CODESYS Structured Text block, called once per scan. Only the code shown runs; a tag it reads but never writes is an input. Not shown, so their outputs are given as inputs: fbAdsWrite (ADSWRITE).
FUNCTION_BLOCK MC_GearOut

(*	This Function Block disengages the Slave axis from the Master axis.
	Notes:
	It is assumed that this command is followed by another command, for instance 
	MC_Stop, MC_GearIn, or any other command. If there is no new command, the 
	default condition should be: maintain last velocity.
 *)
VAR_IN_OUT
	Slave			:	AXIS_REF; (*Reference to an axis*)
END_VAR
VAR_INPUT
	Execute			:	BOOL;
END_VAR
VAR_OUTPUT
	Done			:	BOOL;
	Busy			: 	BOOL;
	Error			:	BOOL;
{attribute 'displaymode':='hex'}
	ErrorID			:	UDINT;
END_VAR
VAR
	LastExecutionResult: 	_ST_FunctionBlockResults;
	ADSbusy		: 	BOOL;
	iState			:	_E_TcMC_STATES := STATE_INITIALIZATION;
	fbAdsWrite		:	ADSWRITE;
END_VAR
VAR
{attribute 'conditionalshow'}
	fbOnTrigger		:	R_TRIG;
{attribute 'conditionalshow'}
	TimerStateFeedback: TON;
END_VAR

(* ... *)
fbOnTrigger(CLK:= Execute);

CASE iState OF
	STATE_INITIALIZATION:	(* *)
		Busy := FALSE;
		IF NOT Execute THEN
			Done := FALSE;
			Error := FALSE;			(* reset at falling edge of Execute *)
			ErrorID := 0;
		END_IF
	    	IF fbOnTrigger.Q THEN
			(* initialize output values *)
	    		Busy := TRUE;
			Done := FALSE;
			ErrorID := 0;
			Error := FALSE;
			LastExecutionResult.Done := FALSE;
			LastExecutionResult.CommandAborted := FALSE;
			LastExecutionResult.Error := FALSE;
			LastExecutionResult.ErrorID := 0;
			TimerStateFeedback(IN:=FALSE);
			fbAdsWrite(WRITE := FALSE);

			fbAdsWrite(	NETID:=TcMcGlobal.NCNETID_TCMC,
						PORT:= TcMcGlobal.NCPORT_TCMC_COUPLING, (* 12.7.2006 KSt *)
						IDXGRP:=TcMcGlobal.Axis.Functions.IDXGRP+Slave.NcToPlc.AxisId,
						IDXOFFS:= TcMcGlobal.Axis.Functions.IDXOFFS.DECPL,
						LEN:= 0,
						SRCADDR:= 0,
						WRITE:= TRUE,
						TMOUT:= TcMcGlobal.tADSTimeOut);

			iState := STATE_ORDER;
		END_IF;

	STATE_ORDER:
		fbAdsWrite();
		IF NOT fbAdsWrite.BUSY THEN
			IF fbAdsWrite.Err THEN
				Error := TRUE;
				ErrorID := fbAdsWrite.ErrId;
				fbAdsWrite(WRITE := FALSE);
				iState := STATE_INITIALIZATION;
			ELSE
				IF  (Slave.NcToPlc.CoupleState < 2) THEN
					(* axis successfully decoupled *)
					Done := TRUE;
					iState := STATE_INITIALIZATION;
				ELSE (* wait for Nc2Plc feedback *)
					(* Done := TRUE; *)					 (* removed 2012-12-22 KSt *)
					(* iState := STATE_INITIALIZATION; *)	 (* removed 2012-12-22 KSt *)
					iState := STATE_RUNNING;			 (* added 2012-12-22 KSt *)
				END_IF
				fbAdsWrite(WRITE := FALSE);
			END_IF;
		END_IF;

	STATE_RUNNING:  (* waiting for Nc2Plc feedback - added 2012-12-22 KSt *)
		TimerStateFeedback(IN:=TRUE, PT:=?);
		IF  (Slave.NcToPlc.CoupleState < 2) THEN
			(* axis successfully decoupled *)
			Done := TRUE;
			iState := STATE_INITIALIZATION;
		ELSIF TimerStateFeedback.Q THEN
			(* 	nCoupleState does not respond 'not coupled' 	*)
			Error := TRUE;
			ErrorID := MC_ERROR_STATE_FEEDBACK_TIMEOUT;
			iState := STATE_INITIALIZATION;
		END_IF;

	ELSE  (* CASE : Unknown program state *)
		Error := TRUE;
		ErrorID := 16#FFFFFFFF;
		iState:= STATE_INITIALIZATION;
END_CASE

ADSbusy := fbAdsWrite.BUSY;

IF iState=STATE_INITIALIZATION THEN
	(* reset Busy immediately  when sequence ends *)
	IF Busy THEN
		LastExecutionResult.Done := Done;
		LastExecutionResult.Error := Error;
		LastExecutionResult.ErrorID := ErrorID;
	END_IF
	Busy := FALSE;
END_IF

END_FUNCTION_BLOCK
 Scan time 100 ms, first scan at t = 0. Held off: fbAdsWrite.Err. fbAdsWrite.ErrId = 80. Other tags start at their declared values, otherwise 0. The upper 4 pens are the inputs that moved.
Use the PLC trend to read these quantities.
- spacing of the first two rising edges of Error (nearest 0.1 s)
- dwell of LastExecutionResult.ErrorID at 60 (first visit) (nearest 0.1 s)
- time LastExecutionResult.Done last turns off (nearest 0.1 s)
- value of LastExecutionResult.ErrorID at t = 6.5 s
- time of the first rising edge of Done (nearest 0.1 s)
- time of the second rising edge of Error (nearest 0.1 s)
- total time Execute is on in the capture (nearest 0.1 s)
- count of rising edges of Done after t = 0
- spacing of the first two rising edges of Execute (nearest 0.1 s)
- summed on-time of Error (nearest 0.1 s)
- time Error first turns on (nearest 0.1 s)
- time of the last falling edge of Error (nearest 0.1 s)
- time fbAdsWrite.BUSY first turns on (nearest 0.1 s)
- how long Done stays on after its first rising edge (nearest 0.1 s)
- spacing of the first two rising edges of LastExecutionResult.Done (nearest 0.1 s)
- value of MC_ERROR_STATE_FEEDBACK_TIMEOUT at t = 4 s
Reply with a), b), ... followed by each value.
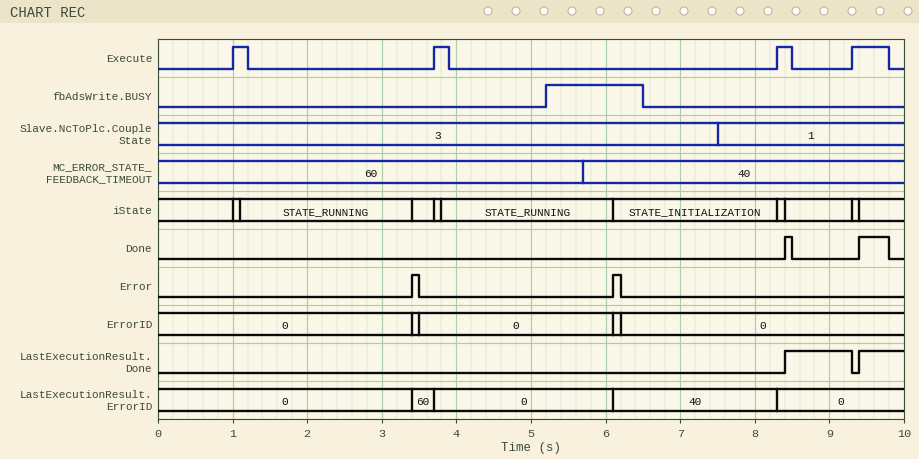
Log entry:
a) 2.7 s
b) 0.3 s
c) 9.3 s
d) 40
e) 8.4 s
f) 6.1 s
g) 1.1 s
h) 2
i) 2.7 s
j) 0.2 s
k) 3.4 s
l) 6.2 s
m) 5.2 s
n) 0.1 s
o) 1.0 s
p) 60
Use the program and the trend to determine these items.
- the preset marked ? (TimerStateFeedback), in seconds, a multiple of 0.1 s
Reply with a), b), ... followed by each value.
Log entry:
a) 2.2 s
